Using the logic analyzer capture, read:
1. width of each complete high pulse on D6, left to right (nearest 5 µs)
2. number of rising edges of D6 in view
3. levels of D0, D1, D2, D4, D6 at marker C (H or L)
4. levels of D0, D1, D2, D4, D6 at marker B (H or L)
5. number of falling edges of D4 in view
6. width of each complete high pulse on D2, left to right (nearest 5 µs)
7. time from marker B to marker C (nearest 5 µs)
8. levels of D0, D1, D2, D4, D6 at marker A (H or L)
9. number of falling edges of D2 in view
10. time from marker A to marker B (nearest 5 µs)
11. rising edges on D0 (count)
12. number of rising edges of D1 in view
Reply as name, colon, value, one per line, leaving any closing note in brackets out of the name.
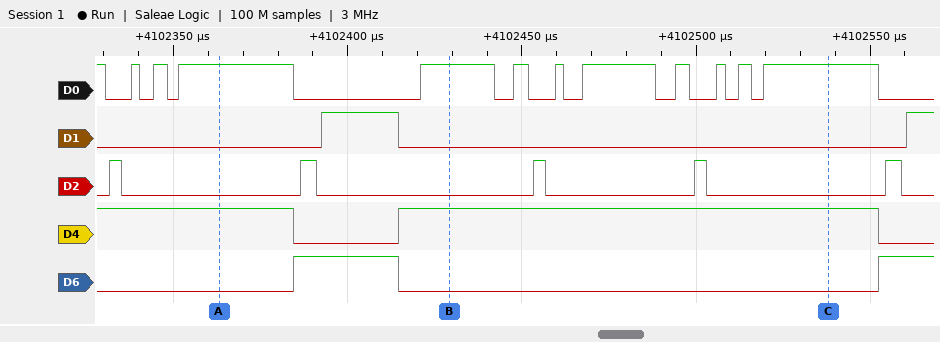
width of each complete high pulse on D6, left to right: 30 µs
number of rising edges of D6 in view: 2
levels of D0, D1, D2, D4, D6 at marker C: D0=H, D1=L, D2=L, D4=H, D6=L
levels of D0, D1, D2, D4, D6 at marker B: D0=H, D1=L, D2=L, D4=H, D6=L
number of falling edges of D4 in view: 2
width of each complete high pulse on D2, left to right: 5 µs, 5 µs, 5 µs, 5 µs, 5 µs
time from marker B to marker C: 110 µs
levels of D0, D1, D2, D4, D6 at marker A: D0=H, D1=L, D2=L, D4=H, D6=L
number of falling edges of D2 in view: 5
time from marker A to marker B: 65 µs
rising edges on D0: 11
number of rising edges of D1 in view: 2
